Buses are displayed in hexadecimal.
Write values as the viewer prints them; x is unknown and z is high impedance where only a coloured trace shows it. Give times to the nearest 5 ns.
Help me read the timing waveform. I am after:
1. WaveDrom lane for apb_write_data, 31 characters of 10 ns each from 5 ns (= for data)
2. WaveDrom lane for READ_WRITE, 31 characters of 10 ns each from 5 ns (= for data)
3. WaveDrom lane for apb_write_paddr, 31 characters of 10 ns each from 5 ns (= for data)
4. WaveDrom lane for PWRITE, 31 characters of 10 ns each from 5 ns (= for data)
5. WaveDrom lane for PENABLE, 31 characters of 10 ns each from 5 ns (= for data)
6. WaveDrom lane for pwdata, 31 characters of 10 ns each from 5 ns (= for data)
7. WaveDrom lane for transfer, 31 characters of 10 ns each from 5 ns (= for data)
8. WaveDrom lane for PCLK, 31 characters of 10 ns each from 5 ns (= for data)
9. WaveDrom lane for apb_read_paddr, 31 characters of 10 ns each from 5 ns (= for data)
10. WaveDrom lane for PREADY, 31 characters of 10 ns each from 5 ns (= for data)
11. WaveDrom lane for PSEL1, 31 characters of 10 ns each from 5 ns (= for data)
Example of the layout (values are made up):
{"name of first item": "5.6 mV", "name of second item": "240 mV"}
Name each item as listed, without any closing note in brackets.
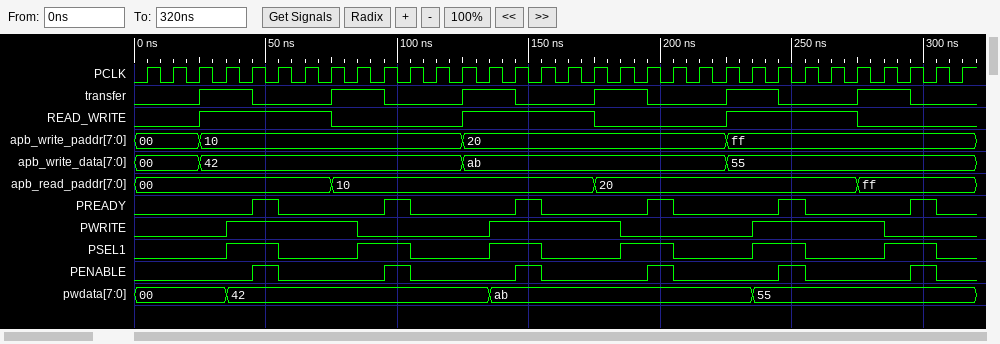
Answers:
{"WaveDrom lane for apb_write_data, 31 characters of 10 ns each from 5 ns": "{name: 'apb_write_data', wave: '=.=.........=.........=........', data: '00 42 ab 55'}", "WaveDrom lane for READ_WRITE, 31 characters of 10 ns each from 5 ns": "{name: 'READ_WRITE', wave: '0.1....0....1....0....1....0...'}", "WaveDrom lane for apb_write_paddr, 31 characters of 10 ns each from 5 ns": "{name: 'apb_write_paddr', wave: '=.=.........=.........=........', data: '00 10 20 ff'}", "WaveDrom lane for PWRITE, 31 characters of 10 ns each from 5 ns": "{name: 'PWRITE', wave: '0..1....0....1....0....1....0..'}", "WaveDrom lane for PENABLE, 31 characters of 10 ns each from 5 ns": "{name: 'PENABLE', wave: '0...10...10...10...10...10...10'}", "WaveDrom lane for pwdata, 31 characters of 10 ns each from 5 ns": "{name: 'pwdata', wave: '=..=.........=.........=.......', data: '00 42 ab 55'}", "WaveDrom lane for transfer, 31 characters of 10 ns each from 5 ns": "{name: 'transfer', wave: '0.1.0..1.0..1.0..1.0..1.0..1.0.'}", "WaveDrom lane for PCLK, 31 characters of 10 ns each from 5 ns": "{name: 'PCLK', wave: 'p..............................'}", "WaveDrom lane for apb_read_paddr, 31 characters of 10 ns each from 5 ns": "{name: 'apb_read_paddr', wave: '=......=.........=.........=...', data: '00 10 20 ff'}", "WaveDrom lane for PREADY, 31 characters of 10 ns each from 5 ns": "{name: 'PREADY', wave: '0...10...10...10...10...10...10'}", "WaveDrom lane for PSEL1, 31 characters of 10 ns each from 5 ns": "{name: 'PSEL1', wave: '0..1.0..1.0..1.0..1.0..1.0..1.0'}"}
